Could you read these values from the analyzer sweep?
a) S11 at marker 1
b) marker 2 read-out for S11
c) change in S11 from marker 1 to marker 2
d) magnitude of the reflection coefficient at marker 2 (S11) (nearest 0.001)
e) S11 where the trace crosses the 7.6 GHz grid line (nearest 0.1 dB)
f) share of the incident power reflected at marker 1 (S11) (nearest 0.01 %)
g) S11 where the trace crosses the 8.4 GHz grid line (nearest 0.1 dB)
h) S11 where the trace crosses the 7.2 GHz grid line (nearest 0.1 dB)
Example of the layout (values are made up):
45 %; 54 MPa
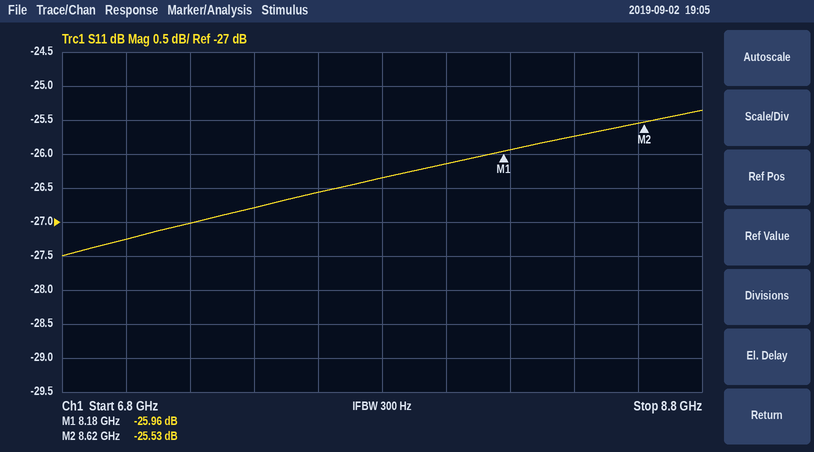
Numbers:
-25.96 dB; -25.53 dB; 0.43 dB; 0.053; -26.6 dB; 0.25 %; -25.7 dB; -27.0 dB
